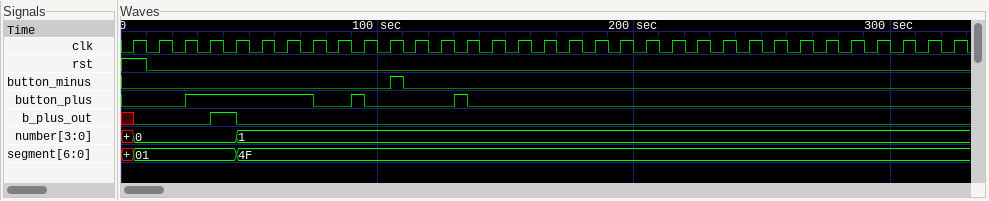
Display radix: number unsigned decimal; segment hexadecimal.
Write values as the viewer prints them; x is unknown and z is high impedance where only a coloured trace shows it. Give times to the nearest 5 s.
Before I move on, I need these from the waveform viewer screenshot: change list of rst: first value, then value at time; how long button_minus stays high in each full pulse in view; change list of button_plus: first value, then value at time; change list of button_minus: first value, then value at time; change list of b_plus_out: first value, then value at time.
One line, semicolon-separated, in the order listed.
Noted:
1, 0 at 10 s; 5 s; 0, 1 at 25 s, 0 at 75 s, 1 at 90 s, 0 at 95 s, 1 at 130 s, 0 at 135 s; 0, 1 at 105 s, 0 at 110 s; x, 0 at 5 s, 1 at 35 s, 0 at 45 s
